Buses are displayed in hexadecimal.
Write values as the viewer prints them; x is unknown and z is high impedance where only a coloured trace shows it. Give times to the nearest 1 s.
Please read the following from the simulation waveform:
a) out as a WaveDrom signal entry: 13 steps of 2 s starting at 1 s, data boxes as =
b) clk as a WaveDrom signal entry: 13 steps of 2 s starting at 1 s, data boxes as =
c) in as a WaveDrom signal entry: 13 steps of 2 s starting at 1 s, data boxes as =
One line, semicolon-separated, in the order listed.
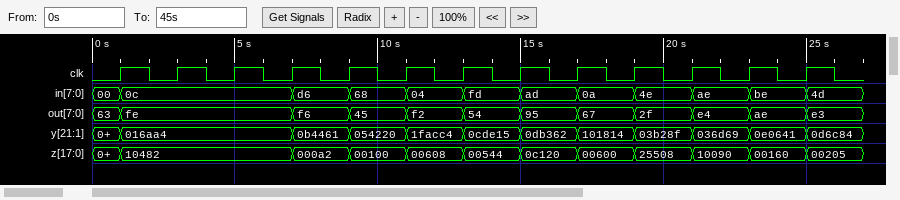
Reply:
{name: 'out', wave: '=..==========', data: 'fe f6 45 f2 54 95 67 2f e4 ae e3'}; {name: 'clk', wave: 'p............'}; {name: 'in', wave: '=..==========', data: '0c d6 68 04 fd ad 0a 4e ae be 4d'}
